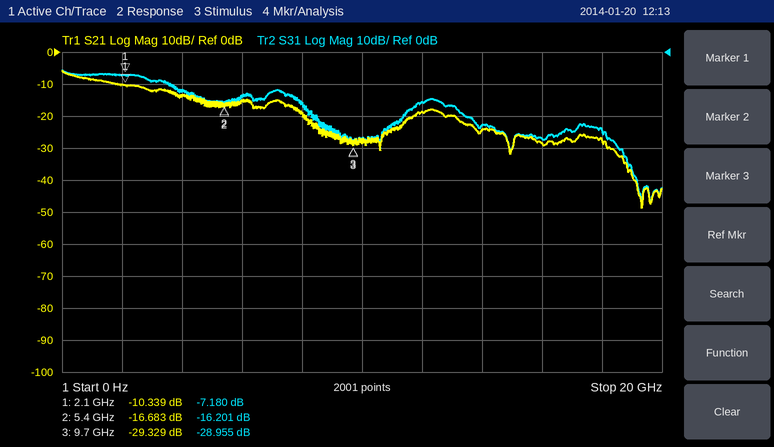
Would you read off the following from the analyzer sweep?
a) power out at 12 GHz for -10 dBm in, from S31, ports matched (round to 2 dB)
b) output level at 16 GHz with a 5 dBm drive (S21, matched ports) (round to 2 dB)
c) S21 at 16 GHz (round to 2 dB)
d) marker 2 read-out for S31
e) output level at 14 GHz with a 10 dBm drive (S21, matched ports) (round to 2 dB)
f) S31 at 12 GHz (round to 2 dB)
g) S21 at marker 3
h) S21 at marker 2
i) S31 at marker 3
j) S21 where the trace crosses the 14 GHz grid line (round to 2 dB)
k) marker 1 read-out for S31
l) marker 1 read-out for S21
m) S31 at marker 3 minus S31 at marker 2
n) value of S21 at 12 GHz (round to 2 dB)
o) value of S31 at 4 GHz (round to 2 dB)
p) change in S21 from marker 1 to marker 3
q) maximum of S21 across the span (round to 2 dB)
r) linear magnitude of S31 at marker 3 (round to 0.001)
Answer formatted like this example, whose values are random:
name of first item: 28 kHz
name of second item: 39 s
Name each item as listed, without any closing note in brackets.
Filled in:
power out at 12 GHz for -10 dBm in, from S31, ports matched: -26 dBm
output level at 16 GHz with a 5 dBm drive (S21, matched ports): -24 dBm
S21 at 16 GHz: -28 dB
marker 2 read-out for S31: -16.201 dB
output level at 14 GHz with a 10 dBm drive (S21, matched ports): -14 dBm
S31 at 12 GHz: -16 dB
S21 at marker 3: -29.329 dB
S21 at marker 2: -16.683 dB
S31 at marker 3: -28.955 dB
S21 where the trace crosses the 14 GHz grid line: -24 dB
marker 1 read-out for S31: -7.180 dB
marker 1 read-out for S21: -10.339 dB
S31 at marker 3 minus S31 at marker 2: -12.754 dB
value of S21 at 12 GHz: -18 dB
value of S31 at 4 GHz: -12 dB
change in S21 from marker 1 to marker 3: -18.990 dB
maximum of S21 across the span: -6 dB
linear magnitude of S31 at marker 3: 0.036
